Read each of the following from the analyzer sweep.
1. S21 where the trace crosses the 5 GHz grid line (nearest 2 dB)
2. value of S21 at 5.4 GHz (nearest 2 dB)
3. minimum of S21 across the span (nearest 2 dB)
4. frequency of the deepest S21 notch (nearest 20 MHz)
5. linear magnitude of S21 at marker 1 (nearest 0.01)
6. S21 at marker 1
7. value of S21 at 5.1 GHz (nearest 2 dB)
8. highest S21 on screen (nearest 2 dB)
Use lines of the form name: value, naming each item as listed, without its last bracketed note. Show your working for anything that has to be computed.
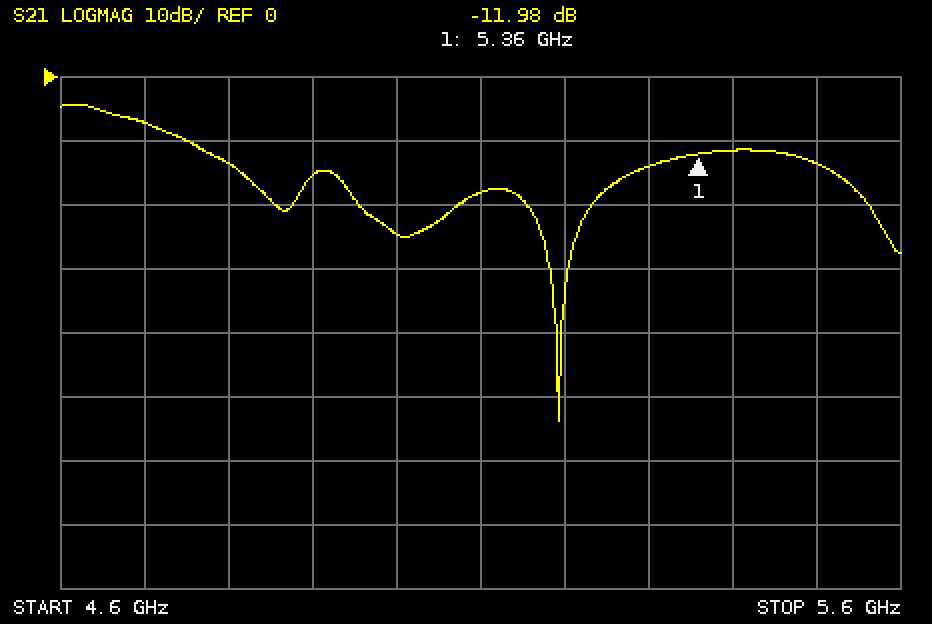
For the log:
S21 where the trace crosses the 5 GHz grid line: -24 dB
value of S21 at 5.4 GHz: -12 dB
minimum of S21 across the span: -54 dB
frequency of the deepest S21 notch: 5.20 GHz
linear magnitude of S21 at marker 1: 10^(-11.98/20) ≈ 0.25
S21 at marker 1: -11.98 dB
value of S21 at 5.1 GHz: -18 dB
highest S21 on screen: -4 dB
